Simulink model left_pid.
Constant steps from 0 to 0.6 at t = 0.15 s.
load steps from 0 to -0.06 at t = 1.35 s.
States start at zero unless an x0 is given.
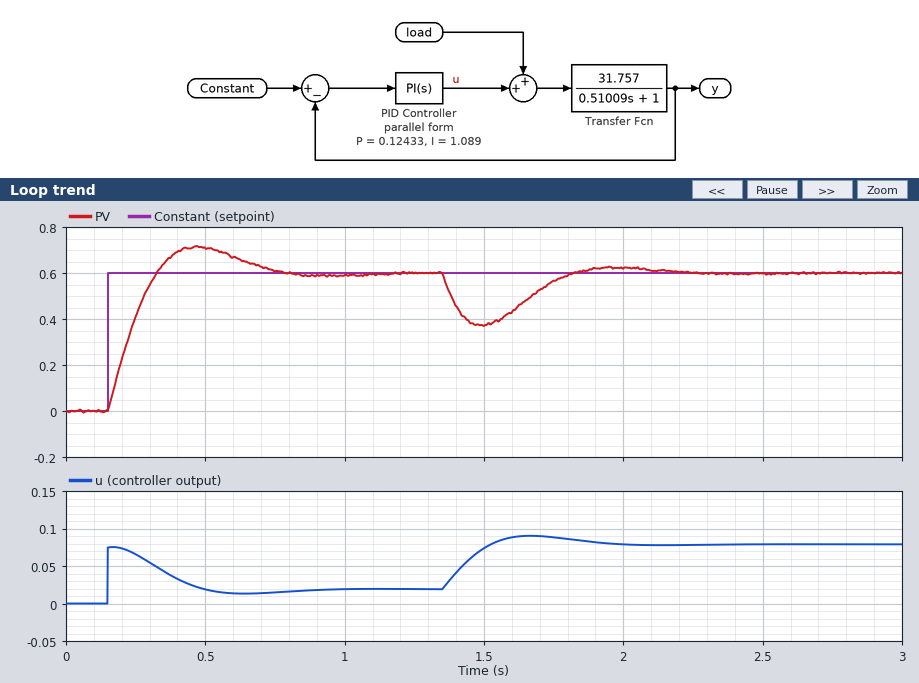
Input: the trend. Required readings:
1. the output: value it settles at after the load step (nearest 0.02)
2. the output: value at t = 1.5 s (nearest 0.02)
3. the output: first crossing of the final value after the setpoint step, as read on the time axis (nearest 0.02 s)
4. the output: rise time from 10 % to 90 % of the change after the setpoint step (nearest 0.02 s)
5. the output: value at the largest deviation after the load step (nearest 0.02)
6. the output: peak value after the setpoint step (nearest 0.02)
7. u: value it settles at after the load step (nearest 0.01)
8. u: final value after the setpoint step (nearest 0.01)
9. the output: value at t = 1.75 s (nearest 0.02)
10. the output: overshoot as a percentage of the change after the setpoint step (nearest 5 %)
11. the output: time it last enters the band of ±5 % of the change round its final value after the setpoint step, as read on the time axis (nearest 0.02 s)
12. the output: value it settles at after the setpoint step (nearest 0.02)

0.60
0.38
0.32 s
0.14 s
0.38
0.72
0.08
0.02
0.56
20 %
0.70 s
0.60
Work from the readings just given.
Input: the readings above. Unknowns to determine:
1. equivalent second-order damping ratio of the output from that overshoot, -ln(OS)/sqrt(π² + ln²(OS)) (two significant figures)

0.46
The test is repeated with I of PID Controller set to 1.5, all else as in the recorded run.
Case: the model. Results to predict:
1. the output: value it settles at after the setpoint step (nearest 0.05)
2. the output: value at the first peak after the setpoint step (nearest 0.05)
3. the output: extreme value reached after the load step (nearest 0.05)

0.60
0.75
0.40
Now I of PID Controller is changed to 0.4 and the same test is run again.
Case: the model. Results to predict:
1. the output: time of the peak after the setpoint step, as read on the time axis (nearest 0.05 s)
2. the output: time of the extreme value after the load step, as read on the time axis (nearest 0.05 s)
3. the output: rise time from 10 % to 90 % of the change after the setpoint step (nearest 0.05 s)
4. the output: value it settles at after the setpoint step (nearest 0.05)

0.70 s
1.55 s
0.20 s
0.60
